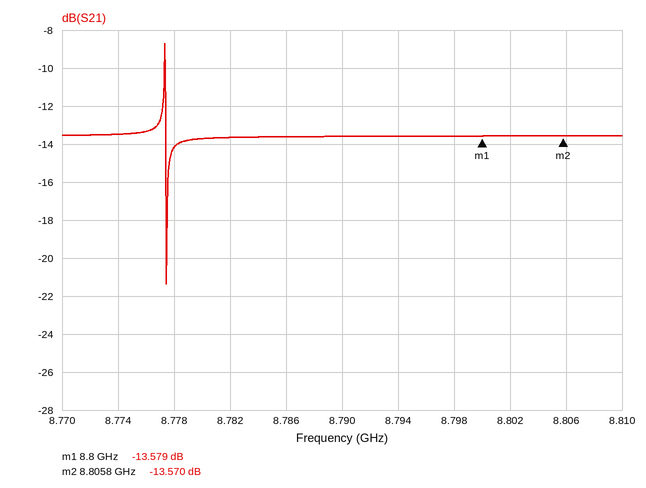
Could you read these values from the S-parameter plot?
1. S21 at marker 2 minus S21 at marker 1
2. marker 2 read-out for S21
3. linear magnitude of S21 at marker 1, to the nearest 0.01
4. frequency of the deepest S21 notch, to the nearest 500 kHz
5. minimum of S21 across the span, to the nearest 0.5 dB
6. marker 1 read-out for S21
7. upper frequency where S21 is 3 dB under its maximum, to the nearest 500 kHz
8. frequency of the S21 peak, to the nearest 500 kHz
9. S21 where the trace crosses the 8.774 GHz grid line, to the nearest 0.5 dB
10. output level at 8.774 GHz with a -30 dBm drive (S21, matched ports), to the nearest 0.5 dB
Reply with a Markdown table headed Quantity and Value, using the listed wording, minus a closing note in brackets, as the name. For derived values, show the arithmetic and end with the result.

| Quantity | Value |
|---|---|
| S21 at marker 2 minus S21 at marker 1 | -13.57 − (-13.579) = 0.009 dB |
| marker 2 read-out for S21 | -13.570 dB |
| linear magnitude of S21 at marker 1, to the nearest 0.01 | 10^(-13.579/20) ≈ 0.21 |
| frequency of the deepest S21 notch, to the nearest 500 kHz | 8.7775 GHz |
| minimum of S21 across the span, to the nearest 0.5 dB | -21.5 dB |
| marker 1 read-out for S21 | -13.579 dB |
| upper frequency where S21 is 3 dB under its maximum, to the nearest 500 kHz | 8.7775 GHz |
| frequency of the S21 peak, to the nearest 500 kHz | 8.7775 GHz |
| S21 where the trace crosses the 8.774 GHz grid line, to the nearest 0.5 dB | -13.5 dB |
| output level at 8.774 GHz with a -30 dBm drive (S21, matched ports), to the nearest 0.5 dB | -30 dBm + (-13.5 dB) = -43.5 dBm |
